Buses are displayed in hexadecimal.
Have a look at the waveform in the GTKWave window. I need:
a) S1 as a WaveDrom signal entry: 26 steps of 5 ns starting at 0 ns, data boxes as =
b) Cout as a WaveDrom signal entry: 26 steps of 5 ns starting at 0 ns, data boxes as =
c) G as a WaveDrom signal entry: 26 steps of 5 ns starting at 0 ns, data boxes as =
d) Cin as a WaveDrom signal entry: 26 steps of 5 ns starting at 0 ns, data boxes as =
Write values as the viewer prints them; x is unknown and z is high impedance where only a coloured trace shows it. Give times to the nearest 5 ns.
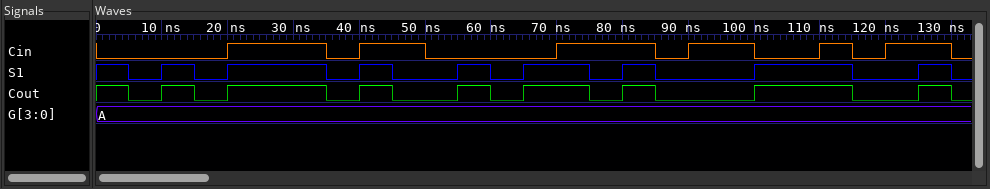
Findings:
{name: 'S1', wave: '10101..010.101.010..1..0.1'}
{name: 'Cout', wave: '10101..010.101.010..1..0.1'}
{name: 'G', wave: '=.........................', data: 'A'}
{name: 'Cin', wave: '0...1..01.0...1..01.0.101.'}
